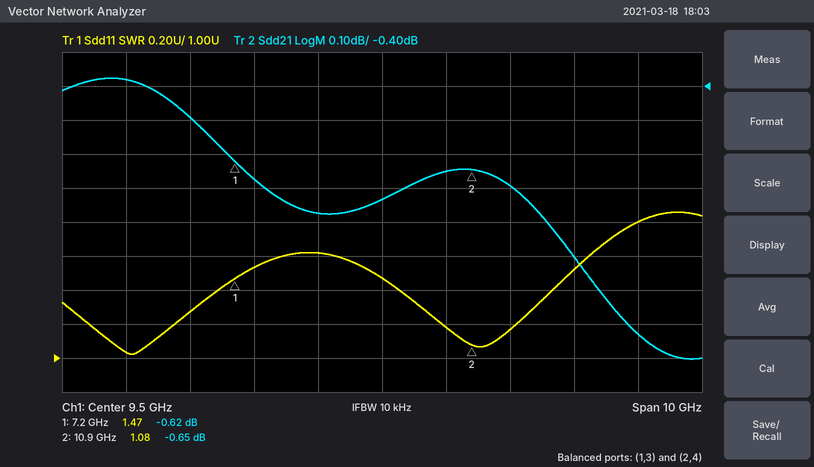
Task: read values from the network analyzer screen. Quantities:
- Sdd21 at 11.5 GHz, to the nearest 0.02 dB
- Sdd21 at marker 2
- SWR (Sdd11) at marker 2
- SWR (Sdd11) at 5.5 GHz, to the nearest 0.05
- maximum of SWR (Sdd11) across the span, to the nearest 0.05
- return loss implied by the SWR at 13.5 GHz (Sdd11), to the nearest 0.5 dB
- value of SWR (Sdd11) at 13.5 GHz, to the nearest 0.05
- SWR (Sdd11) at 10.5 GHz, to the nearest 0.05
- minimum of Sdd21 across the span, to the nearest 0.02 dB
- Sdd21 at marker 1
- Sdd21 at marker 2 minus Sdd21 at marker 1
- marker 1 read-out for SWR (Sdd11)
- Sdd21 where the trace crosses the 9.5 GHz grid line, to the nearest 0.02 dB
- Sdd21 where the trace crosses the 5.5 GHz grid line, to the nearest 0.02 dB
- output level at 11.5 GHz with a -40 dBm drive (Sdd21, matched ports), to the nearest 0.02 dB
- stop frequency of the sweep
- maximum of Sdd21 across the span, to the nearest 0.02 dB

-0.70 dB
-0.65 dB
1.08
1.05
1.85
11.0 dB
1.80
1.20
-1.20 dB
-0.62 dB
-0.03 dB
1.47
-0.74 dB
-0.38 dB
-40.70 dBm
14.5 GHz
-0.38 dB
